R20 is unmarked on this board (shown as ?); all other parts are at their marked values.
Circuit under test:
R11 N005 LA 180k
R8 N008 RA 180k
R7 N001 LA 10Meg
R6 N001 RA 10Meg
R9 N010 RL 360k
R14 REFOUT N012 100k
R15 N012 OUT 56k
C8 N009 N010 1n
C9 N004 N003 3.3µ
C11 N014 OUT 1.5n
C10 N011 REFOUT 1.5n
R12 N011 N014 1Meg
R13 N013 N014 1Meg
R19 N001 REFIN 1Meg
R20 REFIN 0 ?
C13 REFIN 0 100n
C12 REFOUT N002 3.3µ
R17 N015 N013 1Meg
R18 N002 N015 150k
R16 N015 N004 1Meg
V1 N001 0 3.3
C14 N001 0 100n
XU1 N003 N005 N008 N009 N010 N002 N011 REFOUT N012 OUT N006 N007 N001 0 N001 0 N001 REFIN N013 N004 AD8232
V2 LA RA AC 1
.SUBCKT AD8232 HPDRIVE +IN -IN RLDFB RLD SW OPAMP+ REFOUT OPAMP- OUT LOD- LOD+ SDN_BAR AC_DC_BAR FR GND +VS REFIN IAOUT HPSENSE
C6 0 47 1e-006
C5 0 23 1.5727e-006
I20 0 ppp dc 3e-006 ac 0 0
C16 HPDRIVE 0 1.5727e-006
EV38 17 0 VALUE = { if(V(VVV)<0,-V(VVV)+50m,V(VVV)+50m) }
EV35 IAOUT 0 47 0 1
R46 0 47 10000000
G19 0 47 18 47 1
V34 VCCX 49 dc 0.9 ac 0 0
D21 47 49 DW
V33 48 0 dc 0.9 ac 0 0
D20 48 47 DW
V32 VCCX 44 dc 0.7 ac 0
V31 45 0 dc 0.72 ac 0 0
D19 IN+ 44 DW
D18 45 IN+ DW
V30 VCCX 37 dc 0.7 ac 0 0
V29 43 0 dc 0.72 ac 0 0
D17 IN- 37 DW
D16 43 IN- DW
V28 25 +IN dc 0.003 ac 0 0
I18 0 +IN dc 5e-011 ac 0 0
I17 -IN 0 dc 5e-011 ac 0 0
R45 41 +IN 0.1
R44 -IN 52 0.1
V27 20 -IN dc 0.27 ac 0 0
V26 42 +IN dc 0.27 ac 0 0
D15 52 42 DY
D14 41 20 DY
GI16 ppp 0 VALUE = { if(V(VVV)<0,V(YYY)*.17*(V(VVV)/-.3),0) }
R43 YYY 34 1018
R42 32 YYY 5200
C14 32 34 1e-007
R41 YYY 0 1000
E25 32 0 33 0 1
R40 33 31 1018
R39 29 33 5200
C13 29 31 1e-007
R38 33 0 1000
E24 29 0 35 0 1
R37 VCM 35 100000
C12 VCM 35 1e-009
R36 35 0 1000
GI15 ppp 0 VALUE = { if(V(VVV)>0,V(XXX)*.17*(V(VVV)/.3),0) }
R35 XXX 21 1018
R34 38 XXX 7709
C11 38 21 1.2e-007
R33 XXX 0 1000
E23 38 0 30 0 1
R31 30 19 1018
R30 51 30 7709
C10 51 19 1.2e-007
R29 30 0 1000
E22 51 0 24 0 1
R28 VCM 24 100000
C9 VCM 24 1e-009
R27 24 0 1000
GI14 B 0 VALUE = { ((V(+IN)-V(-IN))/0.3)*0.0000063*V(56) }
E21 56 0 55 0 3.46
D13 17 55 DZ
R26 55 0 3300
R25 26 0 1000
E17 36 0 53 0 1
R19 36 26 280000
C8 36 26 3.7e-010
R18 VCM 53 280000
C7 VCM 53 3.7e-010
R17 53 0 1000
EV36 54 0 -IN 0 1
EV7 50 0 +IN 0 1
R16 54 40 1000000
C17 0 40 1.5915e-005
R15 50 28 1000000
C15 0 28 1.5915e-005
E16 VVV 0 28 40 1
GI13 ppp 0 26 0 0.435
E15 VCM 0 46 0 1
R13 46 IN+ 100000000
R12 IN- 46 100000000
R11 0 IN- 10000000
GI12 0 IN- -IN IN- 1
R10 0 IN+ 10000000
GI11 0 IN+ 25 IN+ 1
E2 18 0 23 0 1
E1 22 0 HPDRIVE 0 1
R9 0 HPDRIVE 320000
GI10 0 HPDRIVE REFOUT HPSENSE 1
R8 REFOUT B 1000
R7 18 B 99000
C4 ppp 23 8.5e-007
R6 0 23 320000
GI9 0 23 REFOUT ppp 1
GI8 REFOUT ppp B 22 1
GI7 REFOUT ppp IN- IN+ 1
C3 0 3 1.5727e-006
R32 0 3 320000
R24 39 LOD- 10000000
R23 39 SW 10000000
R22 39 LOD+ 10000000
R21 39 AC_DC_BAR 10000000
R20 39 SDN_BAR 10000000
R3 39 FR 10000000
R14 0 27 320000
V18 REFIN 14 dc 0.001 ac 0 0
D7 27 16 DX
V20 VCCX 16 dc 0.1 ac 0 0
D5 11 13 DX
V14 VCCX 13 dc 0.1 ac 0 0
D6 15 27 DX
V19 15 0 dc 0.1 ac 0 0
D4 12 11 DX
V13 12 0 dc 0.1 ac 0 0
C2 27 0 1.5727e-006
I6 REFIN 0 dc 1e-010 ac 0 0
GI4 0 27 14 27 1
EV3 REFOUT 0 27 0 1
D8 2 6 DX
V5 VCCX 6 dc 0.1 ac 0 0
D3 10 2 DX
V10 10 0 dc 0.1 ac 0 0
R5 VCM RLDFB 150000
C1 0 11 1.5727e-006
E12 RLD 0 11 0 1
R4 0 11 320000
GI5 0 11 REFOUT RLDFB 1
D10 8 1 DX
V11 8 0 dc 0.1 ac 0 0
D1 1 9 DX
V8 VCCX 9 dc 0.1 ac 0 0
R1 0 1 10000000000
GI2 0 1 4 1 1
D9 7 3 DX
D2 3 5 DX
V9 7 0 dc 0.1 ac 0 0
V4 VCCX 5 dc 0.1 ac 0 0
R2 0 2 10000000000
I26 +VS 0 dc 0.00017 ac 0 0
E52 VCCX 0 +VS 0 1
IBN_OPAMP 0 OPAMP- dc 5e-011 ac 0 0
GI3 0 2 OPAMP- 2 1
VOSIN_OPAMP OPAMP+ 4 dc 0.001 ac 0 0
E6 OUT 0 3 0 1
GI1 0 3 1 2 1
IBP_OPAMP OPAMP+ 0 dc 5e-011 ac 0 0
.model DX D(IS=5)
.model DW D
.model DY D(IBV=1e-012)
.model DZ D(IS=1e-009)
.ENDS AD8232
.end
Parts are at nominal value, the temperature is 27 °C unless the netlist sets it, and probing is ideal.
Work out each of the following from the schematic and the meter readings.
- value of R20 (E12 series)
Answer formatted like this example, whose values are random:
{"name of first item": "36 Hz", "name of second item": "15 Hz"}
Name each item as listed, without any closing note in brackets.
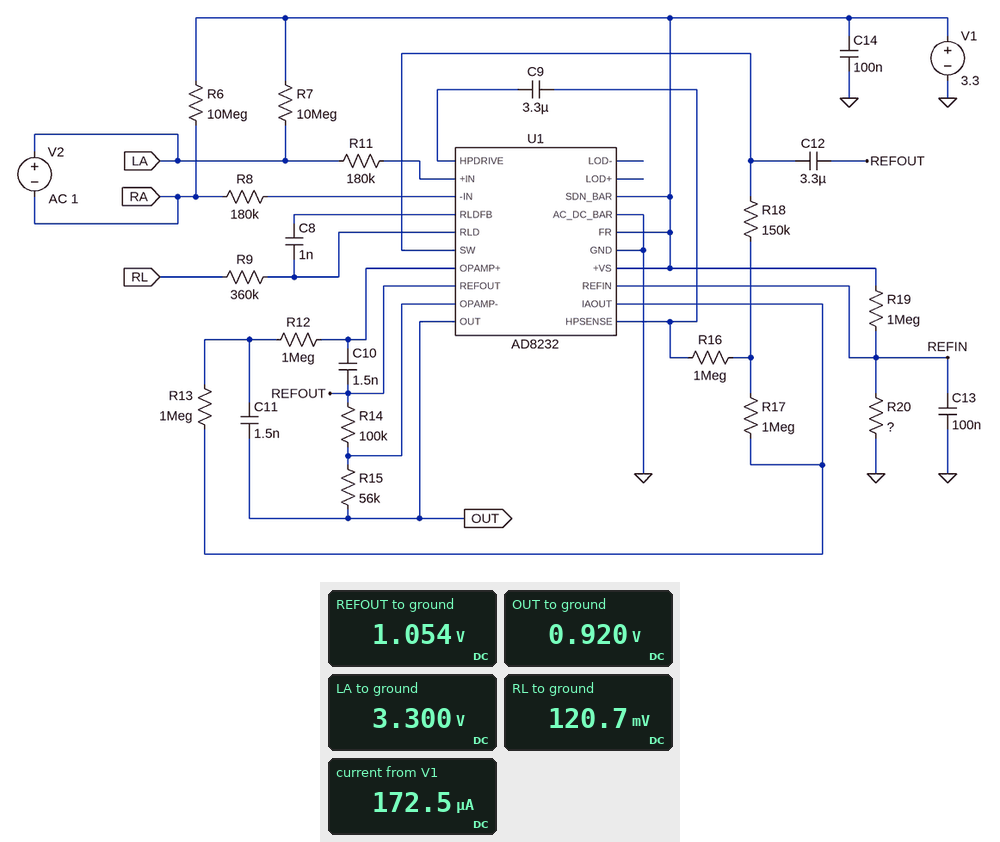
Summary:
{"value of R20": "470 kΩ"}
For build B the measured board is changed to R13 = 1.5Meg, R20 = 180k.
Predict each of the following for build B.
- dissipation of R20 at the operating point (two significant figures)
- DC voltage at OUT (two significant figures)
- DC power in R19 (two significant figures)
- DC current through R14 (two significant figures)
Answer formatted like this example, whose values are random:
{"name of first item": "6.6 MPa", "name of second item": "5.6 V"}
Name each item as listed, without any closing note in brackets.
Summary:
{"dissipation of R20 at the operating point": "1.4 µW", "DC voltage at OUT": "320 mV", "DC power in R19": "7.8 µW", "DC current through R14": "1.2 µA"}
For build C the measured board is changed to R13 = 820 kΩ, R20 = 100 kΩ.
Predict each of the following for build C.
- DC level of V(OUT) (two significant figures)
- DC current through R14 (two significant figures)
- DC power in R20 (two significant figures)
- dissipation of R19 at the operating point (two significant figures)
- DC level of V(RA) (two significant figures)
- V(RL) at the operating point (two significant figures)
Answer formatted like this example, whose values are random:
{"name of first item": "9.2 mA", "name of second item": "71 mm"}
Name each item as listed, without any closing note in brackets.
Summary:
{"DC level of V(OUT)": "230 mV", "DC current through R14": "520 nA", "DC power in R20": "900 nW", "dissipation of R19 at the operating point": "9.0 µW", "DC level of V(RA)": "3.3 V", "V(RL) at the operating point": "110 mV"}
